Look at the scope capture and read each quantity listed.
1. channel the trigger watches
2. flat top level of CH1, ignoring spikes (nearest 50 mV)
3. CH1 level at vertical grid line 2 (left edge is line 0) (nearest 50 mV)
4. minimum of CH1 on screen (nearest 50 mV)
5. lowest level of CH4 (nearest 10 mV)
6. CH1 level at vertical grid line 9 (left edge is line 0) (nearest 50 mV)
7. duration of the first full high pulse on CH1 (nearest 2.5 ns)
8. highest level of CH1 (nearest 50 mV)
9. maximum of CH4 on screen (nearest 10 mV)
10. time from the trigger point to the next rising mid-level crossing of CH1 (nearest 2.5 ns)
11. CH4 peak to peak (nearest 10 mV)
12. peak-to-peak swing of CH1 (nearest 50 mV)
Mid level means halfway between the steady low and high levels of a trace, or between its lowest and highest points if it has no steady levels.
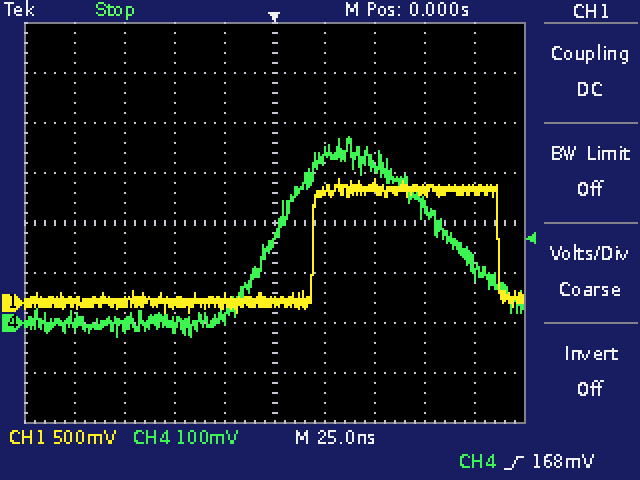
CH4
1.15 V
0 mV
-100 mV
-30 mV
1.15 V
92.5 ns
1.25 V
370 mV
20.0 ns
400 mV
1.35 V
